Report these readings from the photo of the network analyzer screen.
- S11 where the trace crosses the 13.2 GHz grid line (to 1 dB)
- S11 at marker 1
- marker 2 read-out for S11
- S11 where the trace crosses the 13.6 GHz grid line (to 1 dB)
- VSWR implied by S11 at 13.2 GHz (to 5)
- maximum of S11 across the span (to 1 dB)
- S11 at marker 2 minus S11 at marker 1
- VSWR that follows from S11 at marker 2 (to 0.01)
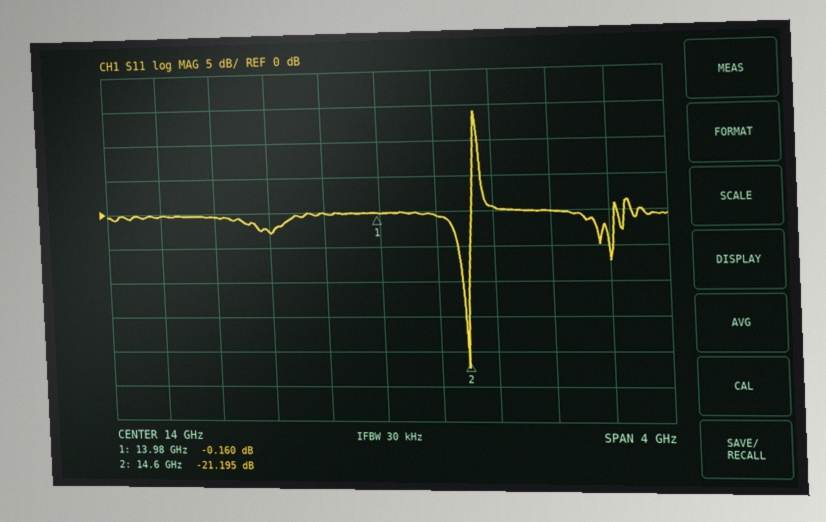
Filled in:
-3 dB
-0.160 dB
-21.195 dB
0 dB
5
14 dB
-21.035 dB
1.19
